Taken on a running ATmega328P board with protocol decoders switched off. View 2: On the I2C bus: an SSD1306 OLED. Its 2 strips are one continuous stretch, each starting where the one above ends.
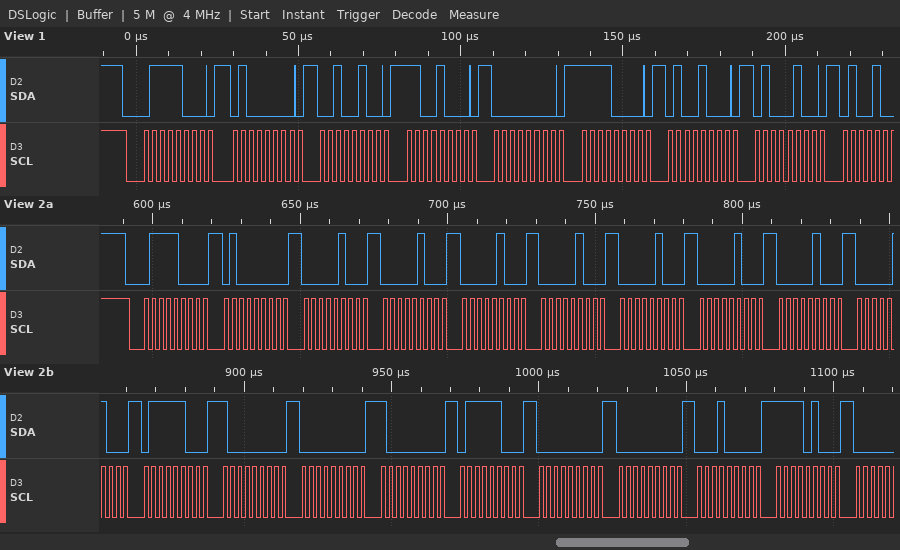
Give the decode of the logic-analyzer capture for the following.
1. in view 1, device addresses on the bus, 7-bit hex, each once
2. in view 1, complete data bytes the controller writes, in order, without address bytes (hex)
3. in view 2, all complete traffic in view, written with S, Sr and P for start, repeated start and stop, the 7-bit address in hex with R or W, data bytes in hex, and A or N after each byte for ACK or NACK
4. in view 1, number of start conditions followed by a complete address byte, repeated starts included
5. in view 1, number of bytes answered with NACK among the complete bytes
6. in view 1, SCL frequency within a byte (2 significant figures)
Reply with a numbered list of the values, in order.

1. 0x3C
2. 40 24 C8 00 F0 48 44
3. S 3CW A 40 A 04 A 04 A 04 A 04 A 04 A 04 A 04 A 04 A 7C A 80 A 00 A 80 A 7C A 00 A 00 A 10 A F4 A
4. 1
5. 0
6. 400 kHz
